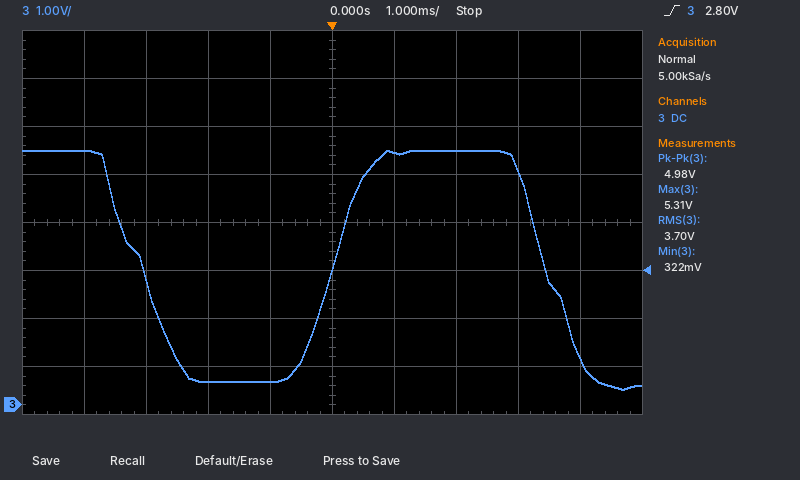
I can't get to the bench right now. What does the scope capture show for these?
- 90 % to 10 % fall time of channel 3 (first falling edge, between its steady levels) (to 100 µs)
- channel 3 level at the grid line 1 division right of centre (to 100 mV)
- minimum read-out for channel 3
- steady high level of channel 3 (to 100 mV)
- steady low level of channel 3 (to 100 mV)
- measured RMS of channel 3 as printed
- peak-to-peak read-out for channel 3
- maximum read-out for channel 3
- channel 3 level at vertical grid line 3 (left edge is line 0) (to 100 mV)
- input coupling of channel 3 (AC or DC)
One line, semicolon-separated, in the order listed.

1.1 ms; 5.3 V; 322 mV; 5.3 V; 500 mV; 3.70 V; 4.98 V; 5.31 V; 500 mV; DC
